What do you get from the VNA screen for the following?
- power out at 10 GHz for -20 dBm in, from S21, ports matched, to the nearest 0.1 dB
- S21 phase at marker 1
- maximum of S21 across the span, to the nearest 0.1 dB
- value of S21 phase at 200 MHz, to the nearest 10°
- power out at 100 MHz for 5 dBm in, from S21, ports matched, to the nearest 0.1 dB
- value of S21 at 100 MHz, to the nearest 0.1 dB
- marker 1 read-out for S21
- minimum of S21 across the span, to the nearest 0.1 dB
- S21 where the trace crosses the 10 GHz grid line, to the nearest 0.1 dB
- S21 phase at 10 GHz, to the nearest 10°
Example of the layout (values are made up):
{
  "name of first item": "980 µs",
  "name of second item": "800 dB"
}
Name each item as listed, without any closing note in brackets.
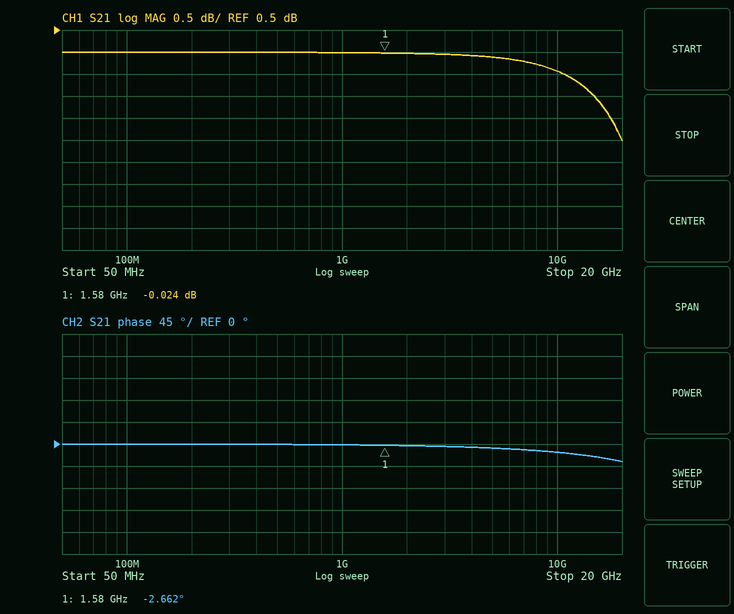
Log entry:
{
  "power out at 10 GHz for -20 dBm in, from S21, ports matched, to the nearest 0.1 dB": "-20.4 dBm",
  "S21 phase at marker 1": "-2.662°",
  "maximum of S21 across the span, to the nearest 0.1 dB": "0.0 dB",
  "value of S21 phase at 200 MHz, to the nearest 10°": "0°",
  "power out at 100 MHz for 5 dBm in, from S21, ports matched, to the nearest 0.1 dB": "5.0 dBm",
  "value of S21 at 100 MHz, to the nearest 0.1 dB": "0.0 dB",
  "marker 1 read-out for S21": "-0.024 dB",
  "minimum of S21 across the span, to the nearest 0.1 dB": "-2.0 dB",
  "S21 where the trace crosses the 10 GHz grid line, to the nearest 0.1 dB": "-0.4 dB",
  "S21 phase at 10 GHz, to the nearest 10°": "-20°"
}
